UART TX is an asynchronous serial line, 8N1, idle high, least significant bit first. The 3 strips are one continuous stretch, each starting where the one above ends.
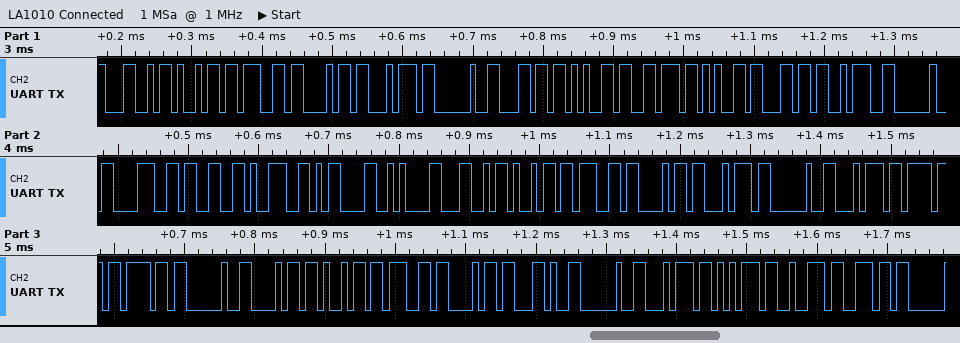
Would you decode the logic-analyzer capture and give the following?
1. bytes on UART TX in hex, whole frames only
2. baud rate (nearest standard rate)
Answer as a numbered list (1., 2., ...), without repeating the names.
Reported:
1. 4C 69 67 68 74 20 6C 65 76 65 6C 3A 20 38 33 39 0D 0A 4C 69 67 68 74 20 74 6F 6F 20 68 69 67 68 2C 20 74 75 72 6E
2. 115200 baud
